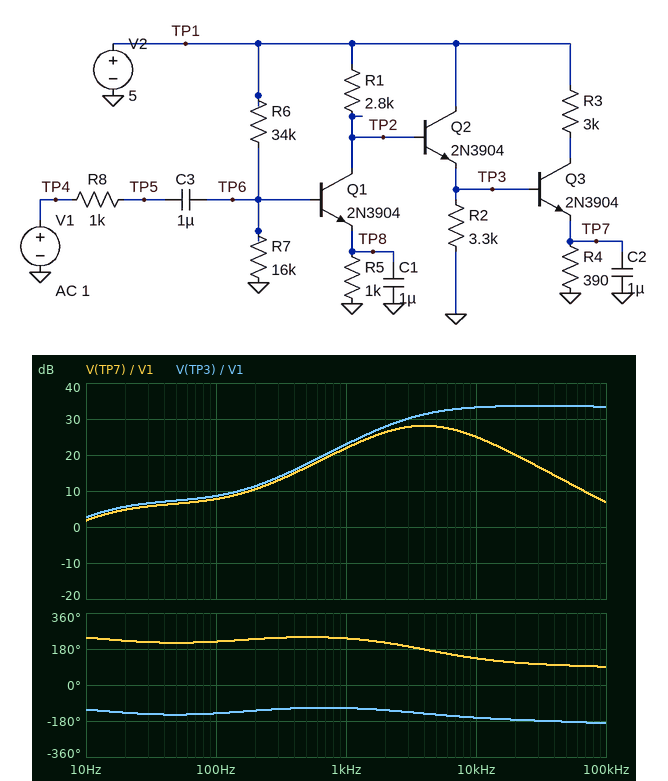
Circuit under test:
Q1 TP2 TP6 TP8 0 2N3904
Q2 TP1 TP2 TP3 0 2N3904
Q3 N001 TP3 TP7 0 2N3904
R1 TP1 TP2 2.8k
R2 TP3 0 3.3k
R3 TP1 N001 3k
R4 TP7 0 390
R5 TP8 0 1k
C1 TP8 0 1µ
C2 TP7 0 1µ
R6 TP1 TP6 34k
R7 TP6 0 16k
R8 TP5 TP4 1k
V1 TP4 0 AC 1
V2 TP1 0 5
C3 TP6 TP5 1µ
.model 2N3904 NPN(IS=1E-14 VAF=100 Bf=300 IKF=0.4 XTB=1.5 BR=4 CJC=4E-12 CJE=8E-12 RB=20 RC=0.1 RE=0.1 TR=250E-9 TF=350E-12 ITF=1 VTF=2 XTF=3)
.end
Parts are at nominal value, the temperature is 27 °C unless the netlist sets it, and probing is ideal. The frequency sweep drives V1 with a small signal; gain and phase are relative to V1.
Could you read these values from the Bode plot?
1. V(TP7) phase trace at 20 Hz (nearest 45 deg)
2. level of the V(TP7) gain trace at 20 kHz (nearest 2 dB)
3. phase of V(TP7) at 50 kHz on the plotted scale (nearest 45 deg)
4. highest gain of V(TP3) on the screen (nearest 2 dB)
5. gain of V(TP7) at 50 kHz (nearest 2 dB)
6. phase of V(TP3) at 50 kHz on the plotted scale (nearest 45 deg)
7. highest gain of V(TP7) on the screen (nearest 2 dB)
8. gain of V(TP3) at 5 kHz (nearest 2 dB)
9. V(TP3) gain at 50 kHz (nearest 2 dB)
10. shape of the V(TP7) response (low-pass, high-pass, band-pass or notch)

225 deg
20 dB
90 deg
34 dB
12 dB
-180 deg
28 dB
32 dB
34 dB
band-pass
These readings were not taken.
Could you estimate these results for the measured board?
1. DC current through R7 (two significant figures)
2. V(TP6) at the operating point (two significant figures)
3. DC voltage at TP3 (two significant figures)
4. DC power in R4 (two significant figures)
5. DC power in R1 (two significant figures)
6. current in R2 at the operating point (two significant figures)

98 µA
1.6 V
1.8 V
2.7 mW
2.4 mW
530 µA
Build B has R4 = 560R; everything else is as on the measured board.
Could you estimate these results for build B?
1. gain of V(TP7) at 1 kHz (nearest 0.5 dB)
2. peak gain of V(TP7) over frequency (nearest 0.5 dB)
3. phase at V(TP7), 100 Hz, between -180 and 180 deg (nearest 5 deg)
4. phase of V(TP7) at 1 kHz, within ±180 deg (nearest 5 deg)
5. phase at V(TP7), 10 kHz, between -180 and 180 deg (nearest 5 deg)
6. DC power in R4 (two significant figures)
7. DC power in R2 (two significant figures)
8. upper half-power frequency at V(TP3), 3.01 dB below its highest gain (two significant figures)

21.5 dB
26.5 dB
-145 deg
-135 deg
130 deg
2.1 mW
960 µW
360 kHz
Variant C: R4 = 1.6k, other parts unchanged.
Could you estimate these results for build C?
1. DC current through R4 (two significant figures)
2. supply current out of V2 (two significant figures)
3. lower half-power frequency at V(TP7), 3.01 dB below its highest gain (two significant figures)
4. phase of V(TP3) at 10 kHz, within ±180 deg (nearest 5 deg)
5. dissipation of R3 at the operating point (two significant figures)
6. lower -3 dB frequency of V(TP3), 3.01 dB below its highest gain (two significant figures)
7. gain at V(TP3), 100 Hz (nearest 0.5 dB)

720 µA
2.3 mA
2.0 kHz
-155 deg
1.6 mW
5.0 kHz
9.0 dB
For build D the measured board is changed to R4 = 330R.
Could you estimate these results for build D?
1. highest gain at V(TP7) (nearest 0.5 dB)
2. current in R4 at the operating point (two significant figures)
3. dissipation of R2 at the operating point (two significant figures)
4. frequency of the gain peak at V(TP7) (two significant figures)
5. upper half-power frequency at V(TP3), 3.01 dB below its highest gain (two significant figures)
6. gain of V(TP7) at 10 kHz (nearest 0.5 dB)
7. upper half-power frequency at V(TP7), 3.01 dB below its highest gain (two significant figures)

28.5 dB
3.0 mA
930 µW
4.2 kHz
450 kHz
26.0 dB
10 kHz
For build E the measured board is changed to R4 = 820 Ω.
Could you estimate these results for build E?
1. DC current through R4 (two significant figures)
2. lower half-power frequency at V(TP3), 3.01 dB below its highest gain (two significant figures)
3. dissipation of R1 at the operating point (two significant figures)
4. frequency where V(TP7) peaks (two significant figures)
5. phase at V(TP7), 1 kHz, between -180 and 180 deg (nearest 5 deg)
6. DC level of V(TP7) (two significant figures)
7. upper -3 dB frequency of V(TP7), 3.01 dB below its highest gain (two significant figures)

1.4 mA
4.6 kHz
2.3 mW
2.7 kHz
-145 deg
1.1 V
7.5 kHz
